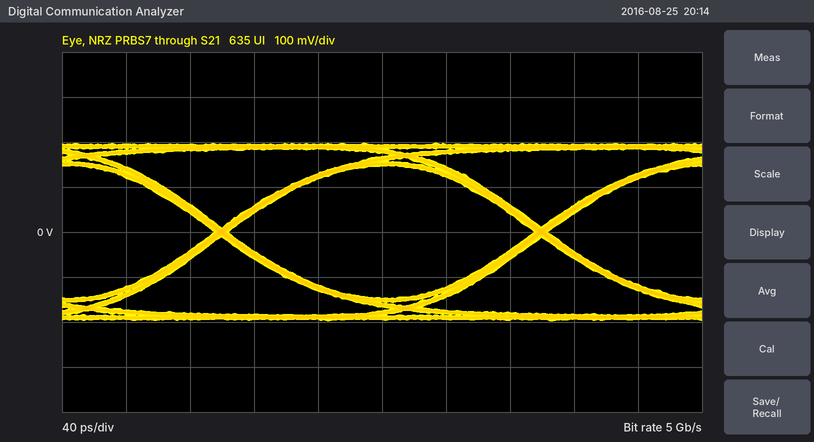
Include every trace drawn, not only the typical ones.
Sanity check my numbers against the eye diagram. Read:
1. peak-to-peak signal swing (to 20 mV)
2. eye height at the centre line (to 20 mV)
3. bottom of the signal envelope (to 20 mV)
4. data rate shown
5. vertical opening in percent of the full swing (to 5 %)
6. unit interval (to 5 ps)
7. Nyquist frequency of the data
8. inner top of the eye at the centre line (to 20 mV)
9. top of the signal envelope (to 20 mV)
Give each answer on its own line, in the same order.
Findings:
400 mV
300 mV
-200 mV
5 Gb/s
75 %
200 ps
2.5 GHz
140 mV
200 mV
